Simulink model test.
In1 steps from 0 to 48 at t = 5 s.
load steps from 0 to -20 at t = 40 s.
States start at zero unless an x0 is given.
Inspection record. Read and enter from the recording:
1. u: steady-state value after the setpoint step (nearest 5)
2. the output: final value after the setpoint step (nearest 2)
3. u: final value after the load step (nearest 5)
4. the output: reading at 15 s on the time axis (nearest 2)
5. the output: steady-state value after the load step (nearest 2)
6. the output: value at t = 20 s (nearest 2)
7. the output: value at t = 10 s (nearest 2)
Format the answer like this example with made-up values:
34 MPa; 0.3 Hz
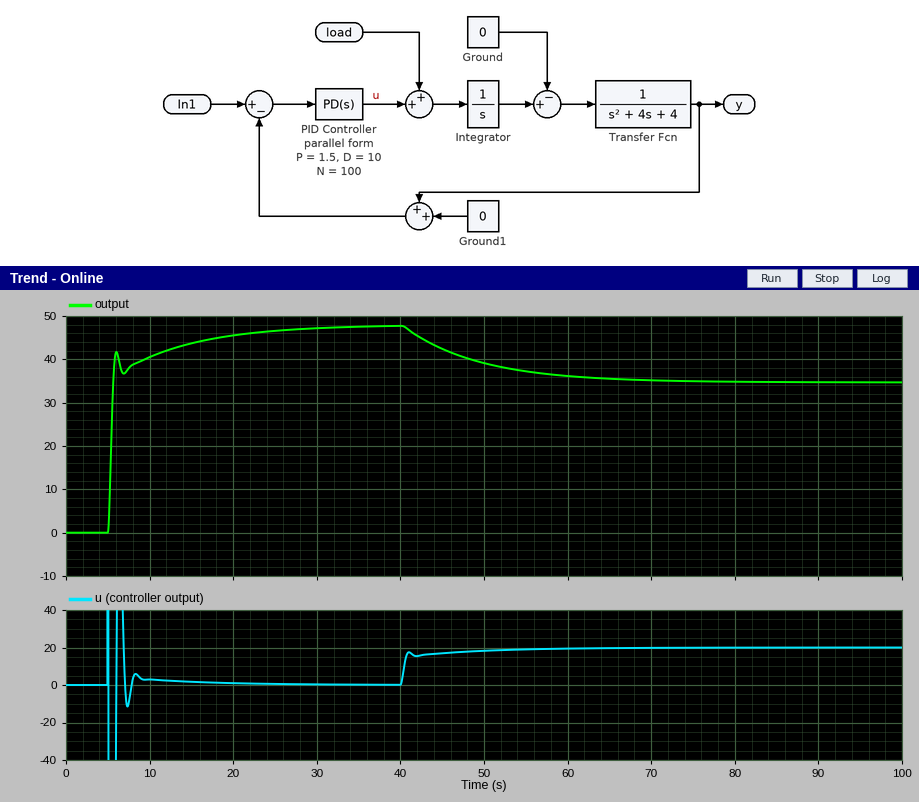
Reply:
0; 48; 20; 44; 34; 46; 40
